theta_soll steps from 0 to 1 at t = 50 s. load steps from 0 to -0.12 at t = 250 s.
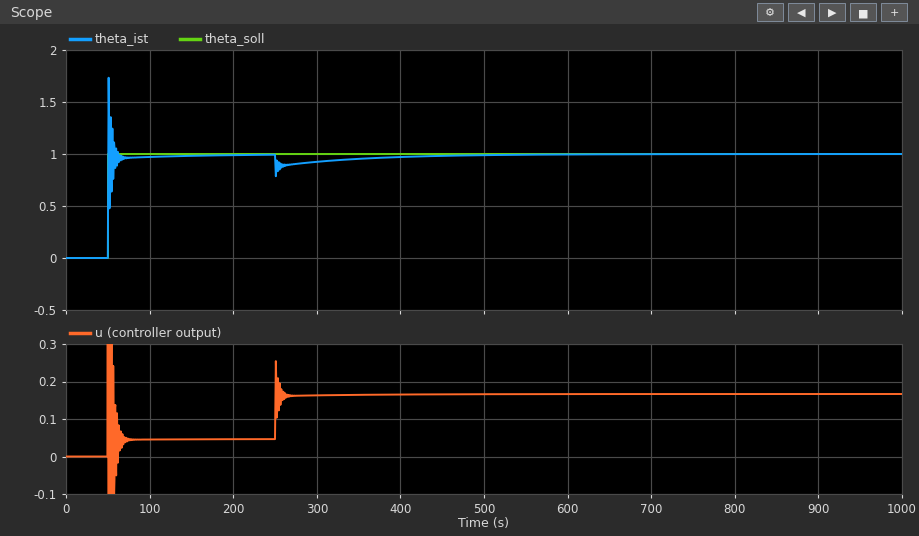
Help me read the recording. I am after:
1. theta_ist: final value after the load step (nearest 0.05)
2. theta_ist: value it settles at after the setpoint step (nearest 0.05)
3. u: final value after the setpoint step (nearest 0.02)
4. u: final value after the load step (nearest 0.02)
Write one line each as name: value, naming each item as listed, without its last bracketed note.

theta_ist: final value after the load step: 1.00
theta_ist: value it settles at after the setpoint step: 1.00
u: final value after the setpoint step: 0.04
u: final value after the load step: 0.16
